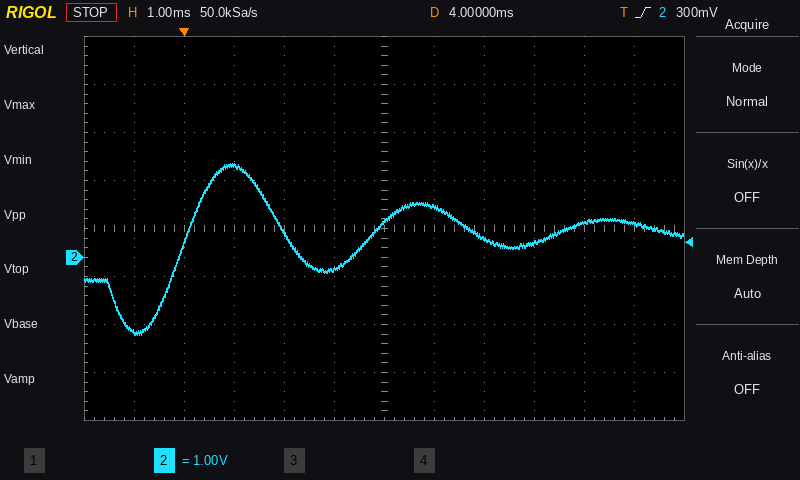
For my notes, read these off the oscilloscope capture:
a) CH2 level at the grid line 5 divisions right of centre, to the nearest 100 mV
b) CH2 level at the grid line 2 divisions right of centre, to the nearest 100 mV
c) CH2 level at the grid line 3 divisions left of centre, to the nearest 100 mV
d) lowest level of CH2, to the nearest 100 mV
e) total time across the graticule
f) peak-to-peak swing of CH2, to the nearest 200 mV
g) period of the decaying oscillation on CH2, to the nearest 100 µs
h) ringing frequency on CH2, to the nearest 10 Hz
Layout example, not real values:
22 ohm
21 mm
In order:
700 mV
400 mV
1.9 V
-1.6 V
12 ms
3.6 V
3.7 ms
270 Hz
